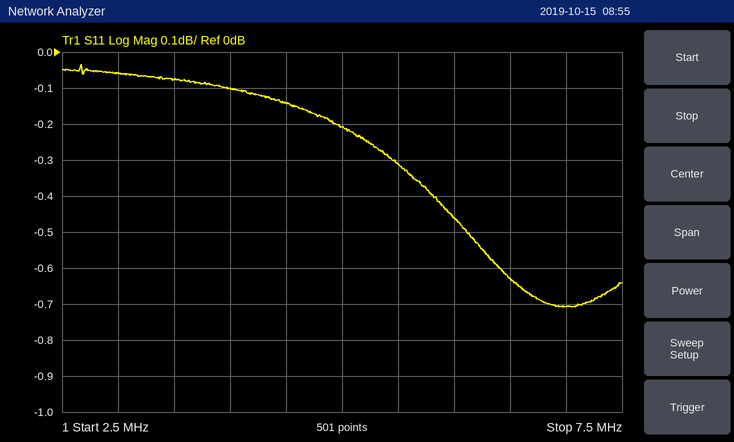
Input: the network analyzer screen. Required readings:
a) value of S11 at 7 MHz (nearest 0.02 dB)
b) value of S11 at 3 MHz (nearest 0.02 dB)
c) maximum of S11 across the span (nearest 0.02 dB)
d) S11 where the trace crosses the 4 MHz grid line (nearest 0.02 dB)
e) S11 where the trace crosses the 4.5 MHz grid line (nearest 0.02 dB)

-0.70 dB
-0.06 dB
-0.04 dB
-0.10 dB
-0.14 dB
